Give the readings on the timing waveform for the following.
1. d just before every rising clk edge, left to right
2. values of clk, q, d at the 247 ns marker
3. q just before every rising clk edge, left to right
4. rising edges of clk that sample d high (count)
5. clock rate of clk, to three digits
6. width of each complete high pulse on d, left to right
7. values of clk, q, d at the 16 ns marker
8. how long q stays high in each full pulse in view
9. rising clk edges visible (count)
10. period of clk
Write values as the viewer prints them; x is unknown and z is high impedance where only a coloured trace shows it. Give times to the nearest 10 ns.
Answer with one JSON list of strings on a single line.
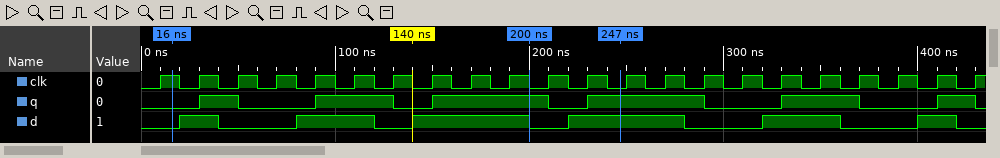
["0 1 0 0 1 1 0 1 1 1 0 1 1 1 0 0 1 1 0 0 1 0", "clk=0, q=1, d=1", "0 0 1 0 0 1 1 0 1 1 1 0 1 1 1 0 0 1 1 0 0 1", "12", "50.0 MHz", "20 ns, 40 ns, 60 ns, 60 ns, 40 ns, 20 ns", "clk=1, q=0, d=0", "20 ns, 40 ns, 60 ns, 60 ns, 40 ns, 20 ns", "22", "20 ns"]
